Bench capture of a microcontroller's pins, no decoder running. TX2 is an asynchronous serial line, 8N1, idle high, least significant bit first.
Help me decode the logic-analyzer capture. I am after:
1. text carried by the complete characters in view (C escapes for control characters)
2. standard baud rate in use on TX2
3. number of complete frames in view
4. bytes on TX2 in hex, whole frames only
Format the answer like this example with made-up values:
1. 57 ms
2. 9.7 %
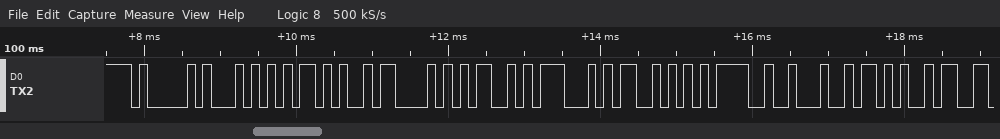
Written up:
1. "AT+CMGS=\"+"
2. 9600 baud
3. 10
4. 41 54 2B 43 4D 47 53 3D 22 2B
